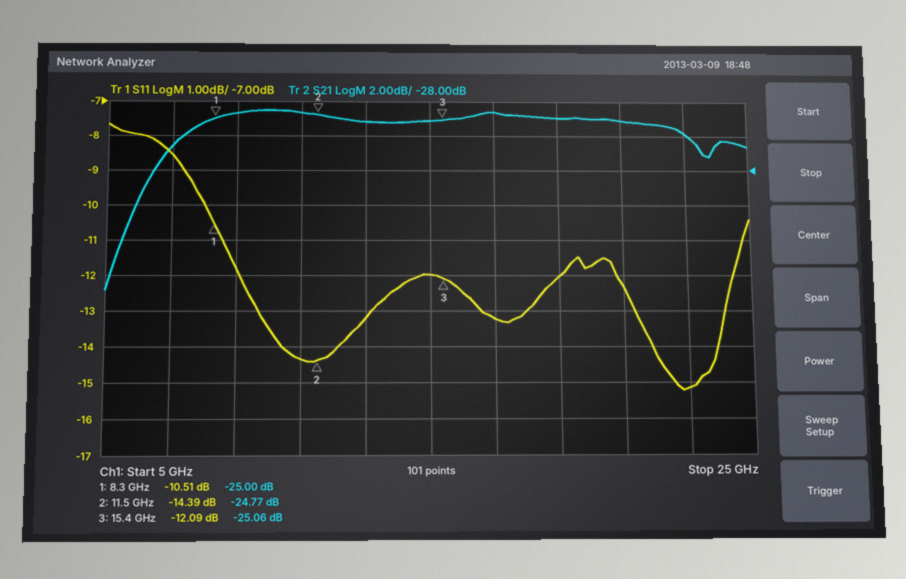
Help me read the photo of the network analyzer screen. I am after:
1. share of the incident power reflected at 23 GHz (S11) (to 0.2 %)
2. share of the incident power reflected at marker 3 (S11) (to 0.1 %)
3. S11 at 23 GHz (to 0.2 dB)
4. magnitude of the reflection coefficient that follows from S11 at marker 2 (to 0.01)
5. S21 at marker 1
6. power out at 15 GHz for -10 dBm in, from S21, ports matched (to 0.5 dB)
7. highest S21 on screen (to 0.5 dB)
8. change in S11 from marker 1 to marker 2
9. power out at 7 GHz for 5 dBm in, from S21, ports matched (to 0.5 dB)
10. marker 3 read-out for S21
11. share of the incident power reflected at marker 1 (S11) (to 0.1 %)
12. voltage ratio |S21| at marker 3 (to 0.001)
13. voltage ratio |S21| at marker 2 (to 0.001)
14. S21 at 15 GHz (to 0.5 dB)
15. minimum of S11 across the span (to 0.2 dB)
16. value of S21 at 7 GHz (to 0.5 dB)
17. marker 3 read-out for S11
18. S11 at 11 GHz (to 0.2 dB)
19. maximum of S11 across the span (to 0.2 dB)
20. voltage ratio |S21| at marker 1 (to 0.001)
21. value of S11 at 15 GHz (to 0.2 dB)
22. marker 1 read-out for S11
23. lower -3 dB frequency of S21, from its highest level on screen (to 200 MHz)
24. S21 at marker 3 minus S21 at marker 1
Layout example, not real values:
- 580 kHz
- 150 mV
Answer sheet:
- 3.0 %
- 6.2 %
- -15.2 dB
- 0.19
- -25.00 dB
- -35.0 dBm
- -24.5 dB
- -3.88 dB
- -21.5 dBm
- -25.06 dB
- 8.9 %
- 0.056
- 0.058
- -25.0 dB
- -15.2 dB
- -26.5 dB
- -12.09 dB
- -14.4 dB
- -7.6 dB
- 0.056
- -12.0 dB
- -10.51 dB
- 6.6 GHz
- -0.06 dB
